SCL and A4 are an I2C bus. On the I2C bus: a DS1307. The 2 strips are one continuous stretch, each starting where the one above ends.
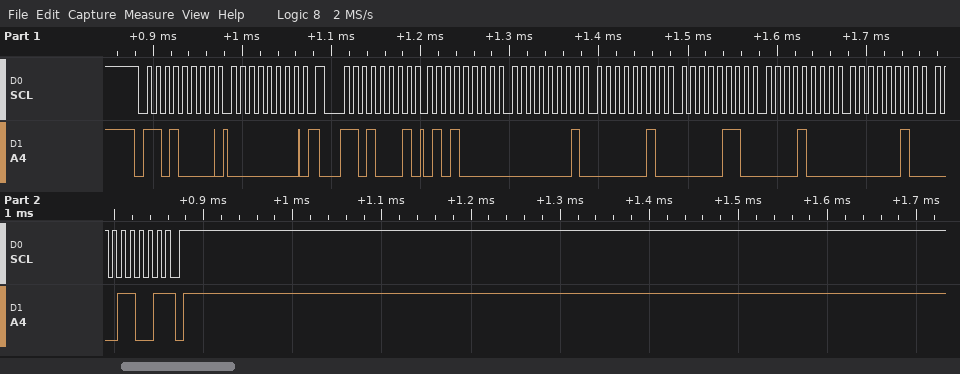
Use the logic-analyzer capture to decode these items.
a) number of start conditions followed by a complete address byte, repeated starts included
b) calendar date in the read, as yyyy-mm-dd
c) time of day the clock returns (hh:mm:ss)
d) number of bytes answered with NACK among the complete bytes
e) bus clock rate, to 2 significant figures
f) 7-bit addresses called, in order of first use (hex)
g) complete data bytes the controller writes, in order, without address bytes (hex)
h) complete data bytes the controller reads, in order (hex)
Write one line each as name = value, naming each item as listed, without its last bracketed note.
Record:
number of start conditions followed by a complete address byte, repeated starts included = 2
calendar date in the read, as yyyy-mm-dd = 2019-02-08
time of day the clock returns = 02:01:50
number of bytes answered with NACK among the complete bytes = 1
bus clock rate, to 2 significant figures = 100 kHz
7-bit addresses called, in order of first use = 0x68
complete data bytes the controller writes, in order, without address bytes = 00
complete data bytes the controller reads, in order = 50 01 02 06 08 02 19
